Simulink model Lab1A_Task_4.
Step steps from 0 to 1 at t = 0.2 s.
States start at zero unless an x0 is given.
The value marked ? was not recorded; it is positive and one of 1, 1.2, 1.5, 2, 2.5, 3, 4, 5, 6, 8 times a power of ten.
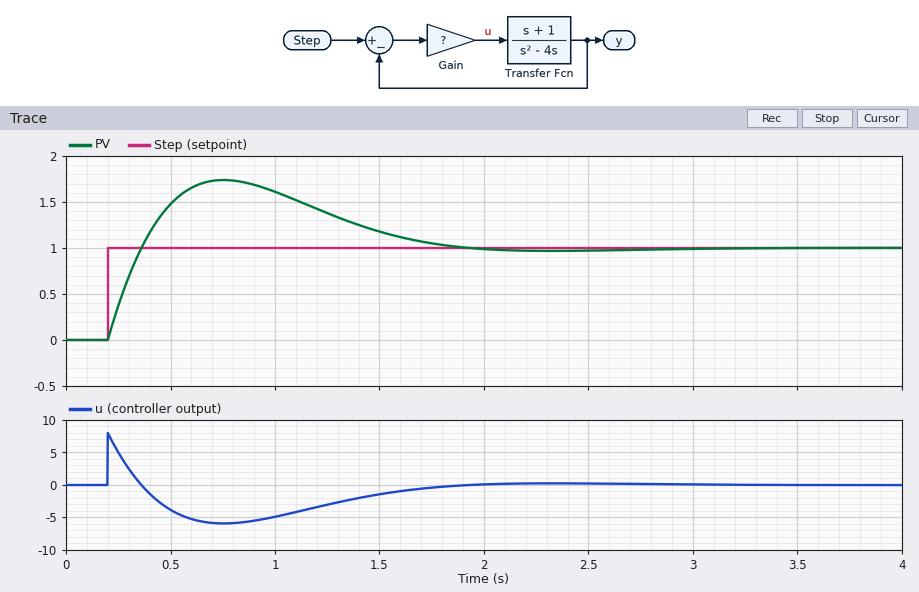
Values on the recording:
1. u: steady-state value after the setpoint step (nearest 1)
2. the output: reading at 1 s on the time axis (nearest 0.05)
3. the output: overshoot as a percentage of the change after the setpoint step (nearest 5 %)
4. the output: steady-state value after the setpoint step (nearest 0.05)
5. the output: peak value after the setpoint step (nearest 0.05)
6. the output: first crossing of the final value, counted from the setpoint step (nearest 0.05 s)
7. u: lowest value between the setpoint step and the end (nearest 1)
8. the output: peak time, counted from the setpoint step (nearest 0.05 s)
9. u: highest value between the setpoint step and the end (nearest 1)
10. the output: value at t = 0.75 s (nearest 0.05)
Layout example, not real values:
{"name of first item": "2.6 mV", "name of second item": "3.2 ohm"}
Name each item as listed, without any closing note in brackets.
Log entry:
{"u: steady-state value after the setpoint step": "0", "the output: reading at 1 s on the time axis": "1.60", "the output: overshoot as a percentage of the change after the setpoint step": "75 %", "the output: steady-state value after the setpoint step": "1.00", "the output: peak value after the setpoint step": "1.75", "the output: first crossing of the final value, counted from the setpoint step": "0.15 s", "u: lowest value between the setpoint step and the end": "-6", "the output: peak time, counted from the setpoint step": "0.55 s", "u: highest value between the setpoint step and the end": "8", "the output: value at t = 0.75 s": "1.75"}
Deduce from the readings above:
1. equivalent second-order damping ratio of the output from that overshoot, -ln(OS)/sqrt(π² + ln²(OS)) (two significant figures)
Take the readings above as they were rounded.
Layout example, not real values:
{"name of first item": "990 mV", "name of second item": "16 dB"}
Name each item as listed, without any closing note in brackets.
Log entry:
{"equivalent second-order damping ratio of the output from that overshoot, -ln(OS)/sqrt(π² + ln²(OS))": "0.091"}
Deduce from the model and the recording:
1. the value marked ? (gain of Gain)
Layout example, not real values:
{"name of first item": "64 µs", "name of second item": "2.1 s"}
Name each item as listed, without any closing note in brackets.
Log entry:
{"the value marked ?": "8"}
